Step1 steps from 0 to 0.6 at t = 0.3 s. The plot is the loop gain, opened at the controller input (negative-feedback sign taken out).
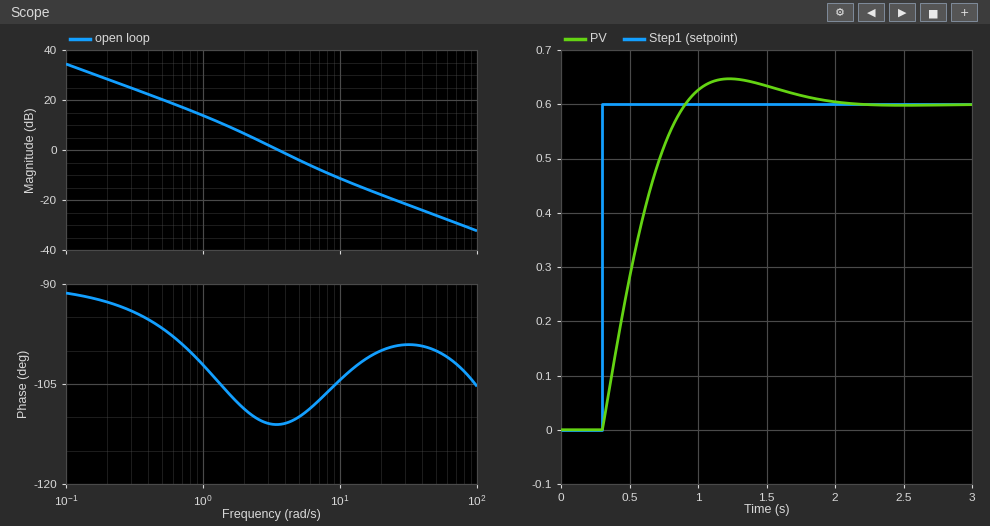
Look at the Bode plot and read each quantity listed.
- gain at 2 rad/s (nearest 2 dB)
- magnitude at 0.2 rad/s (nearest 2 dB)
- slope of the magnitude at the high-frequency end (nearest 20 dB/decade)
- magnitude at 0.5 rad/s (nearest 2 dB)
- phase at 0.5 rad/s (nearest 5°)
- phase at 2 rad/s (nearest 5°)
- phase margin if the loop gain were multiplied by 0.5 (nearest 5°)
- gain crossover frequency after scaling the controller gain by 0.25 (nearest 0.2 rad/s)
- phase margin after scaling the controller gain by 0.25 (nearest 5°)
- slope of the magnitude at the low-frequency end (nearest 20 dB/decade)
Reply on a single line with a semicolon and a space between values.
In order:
6 dB; 28 dB; -20 dB/decade; 20 dB; -95°; -110°; 70°; 1.2 rad/s; 75°; -20 dB/decade
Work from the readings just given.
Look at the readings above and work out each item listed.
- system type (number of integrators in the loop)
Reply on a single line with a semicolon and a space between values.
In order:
1
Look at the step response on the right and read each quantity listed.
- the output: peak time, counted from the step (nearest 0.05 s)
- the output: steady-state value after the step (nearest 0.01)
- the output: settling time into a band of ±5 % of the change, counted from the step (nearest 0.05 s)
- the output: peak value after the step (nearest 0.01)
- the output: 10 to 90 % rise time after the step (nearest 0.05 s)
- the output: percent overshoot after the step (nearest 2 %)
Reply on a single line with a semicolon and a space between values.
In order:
0.95 s; 0.60; 1.25 s; 0.65; 0.45 s; 8 %
